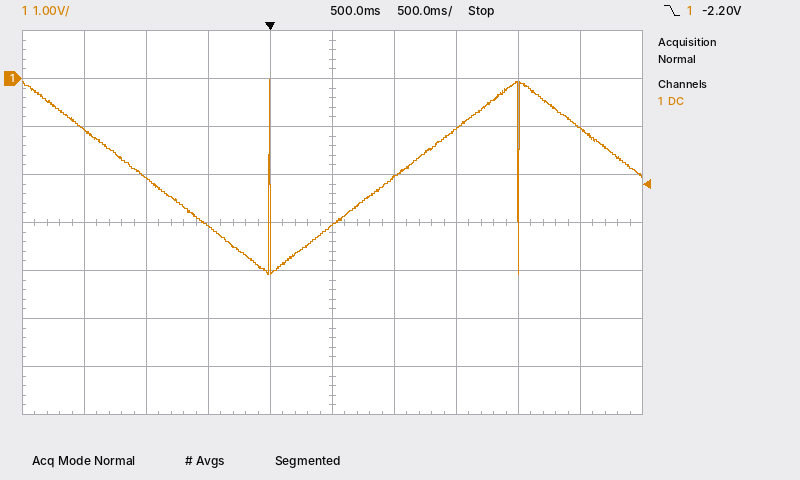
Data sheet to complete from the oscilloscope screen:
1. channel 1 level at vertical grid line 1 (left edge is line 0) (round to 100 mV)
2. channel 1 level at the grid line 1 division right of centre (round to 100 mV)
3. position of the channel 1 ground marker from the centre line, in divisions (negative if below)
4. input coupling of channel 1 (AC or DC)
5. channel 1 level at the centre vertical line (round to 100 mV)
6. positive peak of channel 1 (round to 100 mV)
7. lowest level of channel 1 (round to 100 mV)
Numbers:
-1.1 V
-2.1 V
+3.0 div
DC
-3.1 V
0.0 V
-4.1 V
